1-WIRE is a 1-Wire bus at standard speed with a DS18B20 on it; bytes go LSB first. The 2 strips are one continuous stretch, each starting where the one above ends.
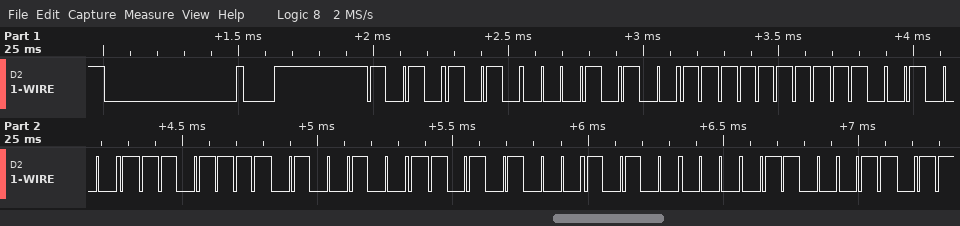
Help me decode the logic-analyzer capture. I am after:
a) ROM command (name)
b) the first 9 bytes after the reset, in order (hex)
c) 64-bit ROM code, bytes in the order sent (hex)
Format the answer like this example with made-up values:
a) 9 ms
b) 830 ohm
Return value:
a) Match ROM
b) 55 28 FF 13 F7 92 15 05 C6
c) 28 FF 13 F7 92 15 05 C6
